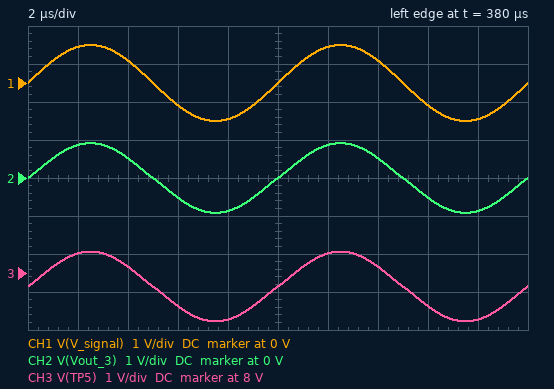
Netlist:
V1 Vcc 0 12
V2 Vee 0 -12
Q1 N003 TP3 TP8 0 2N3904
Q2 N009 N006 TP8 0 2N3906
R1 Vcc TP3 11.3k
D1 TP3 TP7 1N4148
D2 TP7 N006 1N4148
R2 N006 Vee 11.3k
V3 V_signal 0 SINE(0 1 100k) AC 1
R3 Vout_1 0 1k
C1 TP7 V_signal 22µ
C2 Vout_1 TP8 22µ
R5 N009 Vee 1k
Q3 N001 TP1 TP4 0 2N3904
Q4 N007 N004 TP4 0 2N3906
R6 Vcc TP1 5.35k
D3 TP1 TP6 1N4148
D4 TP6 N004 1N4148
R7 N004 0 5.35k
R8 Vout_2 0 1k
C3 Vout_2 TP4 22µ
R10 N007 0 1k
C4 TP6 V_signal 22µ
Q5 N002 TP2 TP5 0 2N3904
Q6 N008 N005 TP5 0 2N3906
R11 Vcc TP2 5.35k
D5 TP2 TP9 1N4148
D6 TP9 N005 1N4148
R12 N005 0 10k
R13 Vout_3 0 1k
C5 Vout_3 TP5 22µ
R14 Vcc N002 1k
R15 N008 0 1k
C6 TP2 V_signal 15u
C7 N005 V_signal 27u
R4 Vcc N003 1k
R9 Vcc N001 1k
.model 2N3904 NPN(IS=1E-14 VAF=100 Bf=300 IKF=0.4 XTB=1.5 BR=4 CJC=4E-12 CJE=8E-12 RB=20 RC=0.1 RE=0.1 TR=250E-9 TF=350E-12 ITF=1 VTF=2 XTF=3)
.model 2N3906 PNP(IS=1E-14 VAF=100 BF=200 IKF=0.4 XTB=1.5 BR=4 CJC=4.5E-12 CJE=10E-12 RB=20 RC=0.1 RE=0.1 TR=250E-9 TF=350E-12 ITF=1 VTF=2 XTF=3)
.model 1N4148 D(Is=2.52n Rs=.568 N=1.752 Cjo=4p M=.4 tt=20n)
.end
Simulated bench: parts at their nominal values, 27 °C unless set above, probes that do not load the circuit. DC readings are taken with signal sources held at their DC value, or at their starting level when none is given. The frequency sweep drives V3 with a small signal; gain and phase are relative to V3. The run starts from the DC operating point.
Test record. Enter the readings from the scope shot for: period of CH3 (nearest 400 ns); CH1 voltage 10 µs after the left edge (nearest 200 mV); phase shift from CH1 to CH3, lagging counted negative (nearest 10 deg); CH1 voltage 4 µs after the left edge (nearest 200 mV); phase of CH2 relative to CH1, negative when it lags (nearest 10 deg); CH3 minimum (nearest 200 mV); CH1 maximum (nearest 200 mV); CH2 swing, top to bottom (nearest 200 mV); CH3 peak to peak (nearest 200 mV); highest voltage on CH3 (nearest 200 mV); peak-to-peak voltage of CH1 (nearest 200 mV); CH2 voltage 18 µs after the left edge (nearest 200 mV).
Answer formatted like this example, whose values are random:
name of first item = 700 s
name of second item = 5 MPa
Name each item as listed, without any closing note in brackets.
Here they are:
period of CH3 = 10.0 µs
CH1 voltage 10 µs after the left edge = 0 V
phase shift from CH1 to CH3, lagging counted negative = 0 deg
CH1 voltage 4 µs after the left edge = 600 mV
phase of CH2 relative to CH1, negative when it lags = 0 deg
CH3 minimum = 6.8 V
CH1 maximum = 1.0 V
CH2 swing, top to bottom = 1.8 V
CH3 peak to peak = 1.8 V
highest voltage on CH3 = 8.6 V
peak-to-peak voltage of CH1 = 2.0 V
CH2 voltage 18 µs after the left edge = -800 mV
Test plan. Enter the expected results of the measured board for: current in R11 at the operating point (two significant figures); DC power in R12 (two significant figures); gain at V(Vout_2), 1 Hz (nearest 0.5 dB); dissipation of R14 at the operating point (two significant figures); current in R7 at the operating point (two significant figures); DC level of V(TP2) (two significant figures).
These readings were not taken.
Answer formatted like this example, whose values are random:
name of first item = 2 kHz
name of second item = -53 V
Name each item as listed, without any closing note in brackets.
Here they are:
current in R11 at the operating point = 710 µA
DC power in R12 = 5.0 mW
gain at V(Vout_2), 1 Hz = -26.5 dB
dissipation of R14 at the operating point = 1.4 µW
current in R7 at the operating point = 1.0 mA
DC level of V(TP2) = 8.2 V
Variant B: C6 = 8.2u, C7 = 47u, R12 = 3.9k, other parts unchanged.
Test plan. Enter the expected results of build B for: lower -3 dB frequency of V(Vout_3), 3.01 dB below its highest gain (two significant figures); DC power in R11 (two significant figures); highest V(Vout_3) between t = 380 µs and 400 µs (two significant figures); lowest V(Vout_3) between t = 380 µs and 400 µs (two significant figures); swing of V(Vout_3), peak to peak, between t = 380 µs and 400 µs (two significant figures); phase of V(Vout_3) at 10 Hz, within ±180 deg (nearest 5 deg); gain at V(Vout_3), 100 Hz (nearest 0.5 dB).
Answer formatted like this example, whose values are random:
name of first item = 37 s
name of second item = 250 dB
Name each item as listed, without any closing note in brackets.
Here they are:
lower -3 dB frequency of V(Vout_3), 3.01 dB below its highest gain = 6.6 Hz
DC power in R11 = 7.3 mW
highest V(Vout_3) between t = 380 µs and 400 µs = 940 mV
lowest V(Vout_3) between t = 380 µs and 400 µs = -940 mV
swing of V(Vout_3), peak to peak, between t = 380 µs and 400 µs = 1.9 V
phase of V(Vout_3) at 10 Hz, within ±180 deg = 40 deg
gain at V(Vout_3), 100 Hz = -1.0 dB
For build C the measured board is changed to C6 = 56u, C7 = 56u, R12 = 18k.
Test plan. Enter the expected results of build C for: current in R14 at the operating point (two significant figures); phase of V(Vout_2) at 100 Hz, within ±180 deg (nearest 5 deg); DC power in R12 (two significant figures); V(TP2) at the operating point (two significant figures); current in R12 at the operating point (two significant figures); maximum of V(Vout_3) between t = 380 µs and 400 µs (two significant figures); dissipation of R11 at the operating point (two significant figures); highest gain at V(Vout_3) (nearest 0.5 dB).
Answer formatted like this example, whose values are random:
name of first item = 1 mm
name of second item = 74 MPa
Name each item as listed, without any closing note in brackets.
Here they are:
current in R14 at the operating point = 18 µA
phase of V(Vout_2) at 100 Hz, within ±180 deg = 5 deg
DC power in R12 = 3.9 mW
V(TP2) at the operating point = 9.5 V
current in R12 at the operating point = 470 µA
maximum of V(Vout_3) between t = 380 µs and 400 µs = 900 mV
dissipation of R11 at the operating point = 1.2 mW
highest gain at V(Vout_3) = -4.5 dB
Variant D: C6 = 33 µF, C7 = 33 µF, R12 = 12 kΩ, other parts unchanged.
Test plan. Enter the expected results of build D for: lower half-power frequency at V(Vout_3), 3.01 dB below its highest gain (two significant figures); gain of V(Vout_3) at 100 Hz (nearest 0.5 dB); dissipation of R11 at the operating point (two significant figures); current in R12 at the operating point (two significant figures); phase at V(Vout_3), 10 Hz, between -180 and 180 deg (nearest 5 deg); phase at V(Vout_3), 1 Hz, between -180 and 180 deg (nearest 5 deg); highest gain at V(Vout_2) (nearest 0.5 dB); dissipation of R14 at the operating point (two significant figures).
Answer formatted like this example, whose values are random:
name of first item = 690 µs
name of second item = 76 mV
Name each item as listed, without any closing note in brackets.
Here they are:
lower half-power frequency at V(Vout_3), 3.01 dB below its highest gain = 5.2 Hz
gain of V(Vout_3) at 100 Hz = -3.0 dB
dissipation of R11 at the operating point = 2.1 mW
current in R12 at the operating point = 630 µA
phase at V(Vout_3), 10 Hz, between -180 and 180 deg = 30 deg
phase at V(Vout_3), 1 Hz, between -180 and 180 deg = 110 deg
highest gain at V(Vout_2) = -1.5 dB
dissipation of R14 at the operating point = 920 nW
